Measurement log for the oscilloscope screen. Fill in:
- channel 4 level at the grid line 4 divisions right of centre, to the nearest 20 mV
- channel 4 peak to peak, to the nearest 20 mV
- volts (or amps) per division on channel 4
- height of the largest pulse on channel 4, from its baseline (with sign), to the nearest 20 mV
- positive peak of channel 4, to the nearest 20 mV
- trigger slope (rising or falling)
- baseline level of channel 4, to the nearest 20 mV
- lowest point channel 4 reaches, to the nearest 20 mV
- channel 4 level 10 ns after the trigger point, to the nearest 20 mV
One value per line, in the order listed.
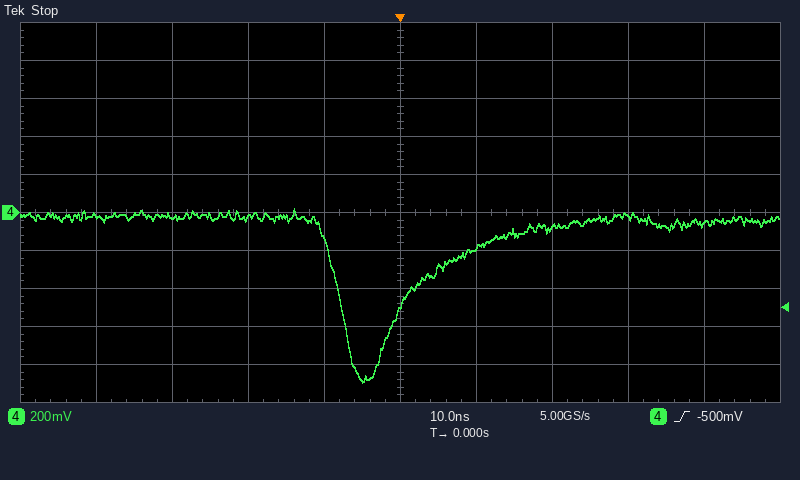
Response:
-60 mV
920 mV
200 mV
-860 mV
20 mV
rising
-40 mV
-900 mV
-180 mV
